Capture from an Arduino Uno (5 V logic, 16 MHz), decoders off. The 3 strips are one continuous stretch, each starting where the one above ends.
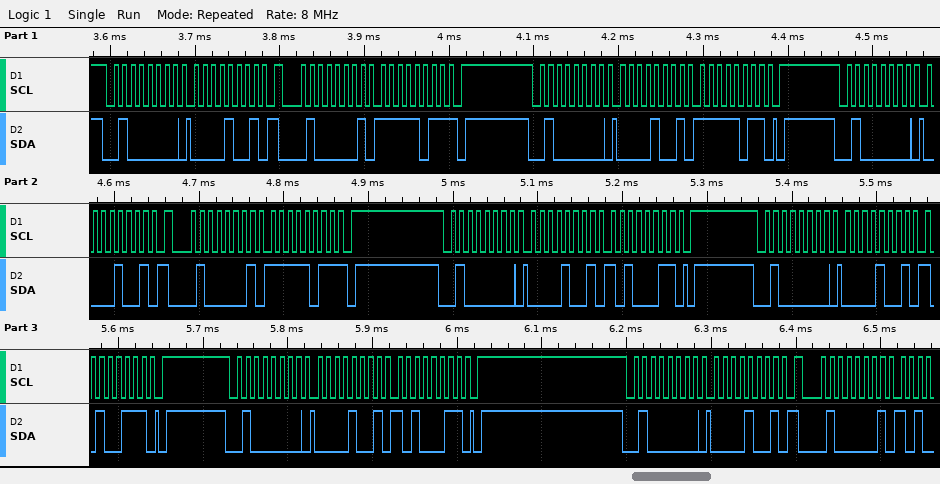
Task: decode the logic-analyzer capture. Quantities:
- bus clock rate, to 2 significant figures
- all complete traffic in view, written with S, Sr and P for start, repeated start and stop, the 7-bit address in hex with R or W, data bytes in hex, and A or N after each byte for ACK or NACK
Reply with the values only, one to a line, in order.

100 kHz
S 20W A 09 A Sr 20R A FB N P S 20W A 09 A FB A P S 20W A 09 A Sr 20R A FB N P S 20W A 09 A A3 A P S 20W A 09 A A7 A P S 20W A 09 A A3 A P S 20W A 09 A Sr 20R A
